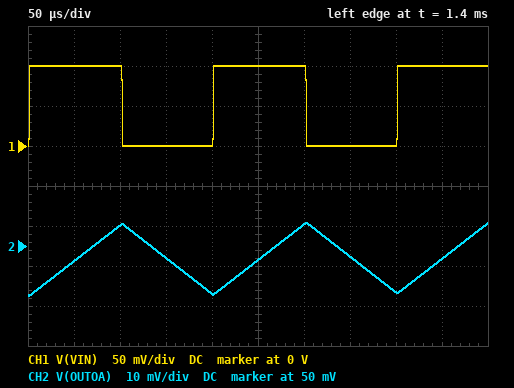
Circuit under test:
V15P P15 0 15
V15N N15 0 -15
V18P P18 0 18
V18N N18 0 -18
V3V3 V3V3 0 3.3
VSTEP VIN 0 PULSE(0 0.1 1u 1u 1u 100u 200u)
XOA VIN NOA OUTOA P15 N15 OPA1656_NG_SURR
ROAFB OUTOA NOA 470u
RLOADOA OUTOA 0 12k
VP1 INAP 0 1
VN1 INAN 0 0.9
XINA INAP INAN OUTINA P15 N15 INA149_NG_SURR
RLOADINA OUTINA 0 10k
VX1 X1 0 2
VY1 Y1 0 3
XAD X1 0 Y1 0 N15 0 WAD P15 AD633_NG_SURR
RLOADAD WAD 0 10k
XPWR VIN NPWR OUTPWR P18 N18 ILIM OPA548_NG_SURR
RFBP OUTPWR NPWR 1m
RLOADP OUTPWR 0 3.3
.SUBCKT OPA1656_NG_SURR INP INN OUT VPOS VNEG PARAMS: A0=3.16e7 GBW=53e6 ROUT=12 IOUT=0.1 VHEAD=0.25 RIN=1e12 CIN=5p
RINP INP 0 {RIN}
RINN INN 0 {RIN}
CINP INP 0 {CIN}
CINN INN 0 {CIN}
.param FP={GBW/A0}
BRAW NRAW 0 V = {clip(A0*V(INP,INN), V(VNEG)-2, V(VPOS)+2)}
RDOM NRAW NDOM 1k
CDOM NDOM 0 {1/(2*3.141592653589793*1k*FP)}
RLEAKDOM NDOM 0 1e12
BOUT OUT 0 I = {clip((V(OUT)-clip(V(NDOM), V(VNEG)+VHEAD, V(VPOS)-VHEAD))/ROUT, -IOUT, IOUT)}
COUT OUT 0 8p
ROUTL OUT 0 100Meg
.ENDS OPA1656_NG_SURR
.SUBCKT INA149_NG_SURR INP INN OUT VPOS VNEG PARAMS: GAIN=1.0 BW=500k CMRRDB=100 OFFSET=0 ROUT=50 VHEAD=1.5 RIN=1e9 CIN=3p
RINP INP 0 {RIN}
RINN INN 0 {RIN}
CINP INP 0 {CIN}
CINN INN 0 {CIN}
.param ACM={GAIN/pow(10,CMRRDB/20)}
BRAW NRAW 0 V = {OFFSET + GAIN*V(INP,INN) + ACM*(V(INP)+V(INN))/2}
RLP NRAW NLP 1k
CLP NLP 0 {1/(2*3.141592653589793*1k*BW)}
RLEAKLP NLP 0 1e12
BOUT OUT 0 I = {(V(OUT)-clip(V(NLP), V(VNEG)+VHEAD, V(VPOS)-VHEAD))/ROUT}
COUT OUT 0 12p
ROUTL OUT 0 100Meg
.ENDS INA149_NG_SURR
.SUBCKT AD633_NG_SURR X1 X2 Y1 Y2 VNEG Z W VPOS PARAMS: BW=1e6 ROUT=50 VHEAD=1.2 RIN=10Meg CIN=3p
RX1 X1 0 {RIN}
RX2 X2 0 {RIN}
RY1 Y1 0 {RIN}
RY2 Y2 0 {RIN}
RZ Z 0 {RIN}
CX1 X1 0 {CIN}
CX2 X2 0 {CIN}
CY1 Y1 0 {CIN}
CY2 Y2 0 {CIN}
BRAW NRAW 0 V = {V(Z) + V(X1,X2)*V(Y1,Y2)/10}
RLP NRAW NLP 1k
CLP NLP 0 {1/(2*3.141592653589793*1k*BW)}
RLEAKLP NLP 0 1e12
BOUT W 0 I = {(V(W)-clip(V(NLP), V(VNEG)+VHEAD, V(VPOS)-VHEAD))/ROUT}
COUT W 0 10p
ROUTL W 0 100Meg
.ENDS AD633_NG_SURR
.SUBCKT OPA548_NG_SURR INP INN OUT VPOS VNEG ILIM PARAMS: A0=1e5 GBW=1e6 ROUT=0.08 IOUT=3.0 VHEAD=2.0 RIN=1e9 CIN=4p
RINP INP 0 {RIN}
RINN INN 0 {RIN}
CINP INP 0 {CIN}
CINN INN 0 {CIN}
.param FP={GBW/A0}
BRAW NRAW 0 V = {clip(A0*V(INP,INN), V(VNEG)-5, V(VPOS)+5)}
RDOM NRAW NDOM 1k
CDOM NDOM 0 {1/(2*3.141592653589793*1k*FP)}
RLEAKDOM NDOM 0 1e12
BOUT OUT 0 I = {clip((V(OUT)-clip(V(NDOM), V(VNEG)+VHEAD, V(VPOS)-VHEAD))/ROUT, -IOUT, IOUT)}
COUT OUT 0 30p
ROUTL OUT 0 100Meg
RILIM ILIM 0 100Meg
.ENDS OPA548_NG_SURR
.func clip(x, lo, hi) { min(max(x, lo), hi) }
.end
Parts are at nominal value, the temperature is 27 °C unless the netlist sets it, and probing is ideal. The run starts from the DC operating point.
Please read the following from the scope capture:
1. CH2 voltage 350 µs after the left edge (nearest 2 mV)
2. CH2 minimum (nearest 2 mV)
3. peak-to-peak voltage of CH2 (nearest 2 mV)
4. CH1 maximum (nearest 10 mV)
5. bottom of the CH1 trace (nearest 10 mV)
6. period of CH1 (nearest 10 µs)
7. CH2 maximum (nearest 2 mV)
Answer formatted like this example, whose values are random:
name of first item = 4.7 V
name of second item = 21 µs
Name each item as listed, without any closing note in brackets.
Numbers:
CH2 voltage 350 µs after the left edge = 48 mV
CH2 minimum = 38 mV
peak-to-peak voltage of CH2 = 18 mV
CH1 maximum = 100 mV
bottom of the CH1 trace = 0 V
period of CH1 = 200 µs
CH2 maximum = 56 mV
